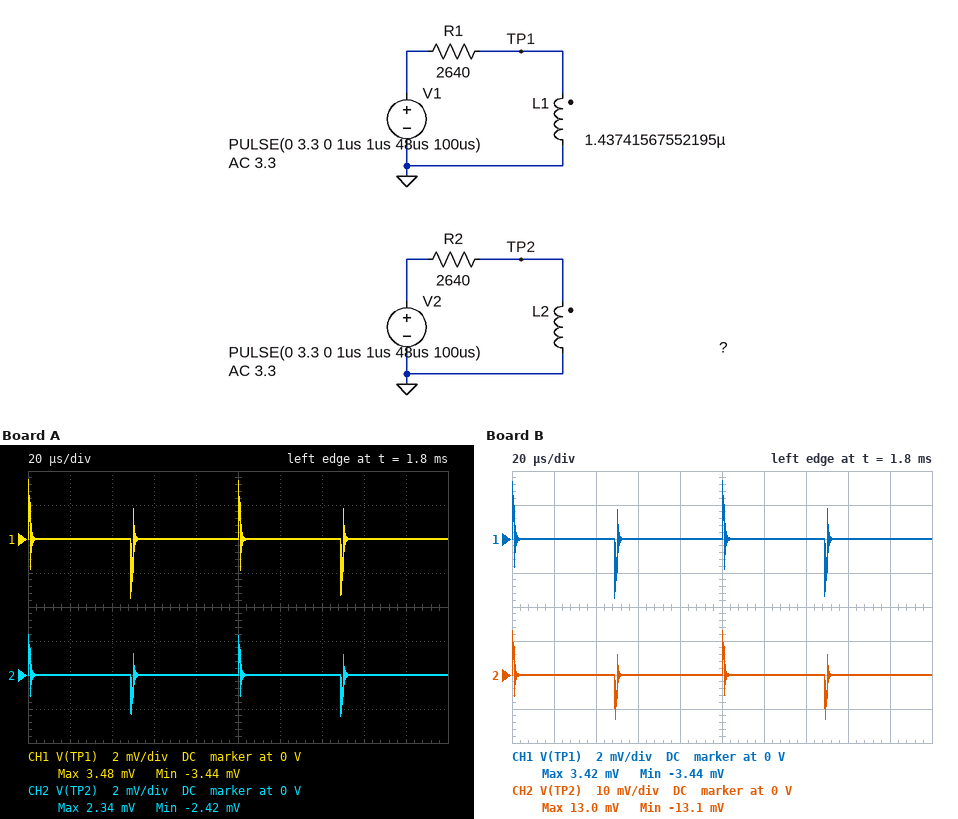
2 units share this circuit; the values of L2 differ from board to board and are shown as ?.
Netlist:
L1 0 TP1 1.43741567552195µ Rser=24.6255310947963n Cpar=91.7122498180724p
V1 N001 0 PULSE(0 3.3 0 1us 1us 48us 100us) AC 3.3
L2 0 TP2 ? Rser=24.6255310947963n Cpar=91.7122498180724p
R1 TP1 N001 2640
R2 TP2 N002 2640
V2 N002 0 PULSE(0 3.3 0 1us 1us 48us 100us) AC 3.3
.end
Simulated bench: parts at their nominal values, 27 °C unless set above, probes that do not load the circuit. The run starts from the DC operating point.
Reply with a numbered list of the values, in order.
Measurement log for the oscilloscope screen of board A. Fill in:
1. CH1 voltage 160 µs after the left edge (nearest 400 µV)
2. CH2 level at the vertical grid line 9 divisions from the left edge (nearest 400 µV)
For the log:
1. 0 V
2. 0 V
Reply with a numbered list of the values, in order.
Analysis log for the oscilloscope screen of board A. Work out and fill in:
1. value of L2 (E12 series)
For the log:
1. 1 µH
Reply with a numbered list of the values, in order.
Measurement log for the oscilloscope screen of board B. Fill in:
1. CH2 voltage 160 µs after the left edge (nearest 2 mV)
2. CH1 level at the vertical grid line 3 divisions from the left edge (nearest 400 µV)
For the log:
1. 0 V
2. 0 V
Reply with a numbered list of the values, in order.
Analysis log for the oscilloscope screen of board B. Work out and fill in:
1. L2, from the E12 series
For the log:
1. 5.6 µH
